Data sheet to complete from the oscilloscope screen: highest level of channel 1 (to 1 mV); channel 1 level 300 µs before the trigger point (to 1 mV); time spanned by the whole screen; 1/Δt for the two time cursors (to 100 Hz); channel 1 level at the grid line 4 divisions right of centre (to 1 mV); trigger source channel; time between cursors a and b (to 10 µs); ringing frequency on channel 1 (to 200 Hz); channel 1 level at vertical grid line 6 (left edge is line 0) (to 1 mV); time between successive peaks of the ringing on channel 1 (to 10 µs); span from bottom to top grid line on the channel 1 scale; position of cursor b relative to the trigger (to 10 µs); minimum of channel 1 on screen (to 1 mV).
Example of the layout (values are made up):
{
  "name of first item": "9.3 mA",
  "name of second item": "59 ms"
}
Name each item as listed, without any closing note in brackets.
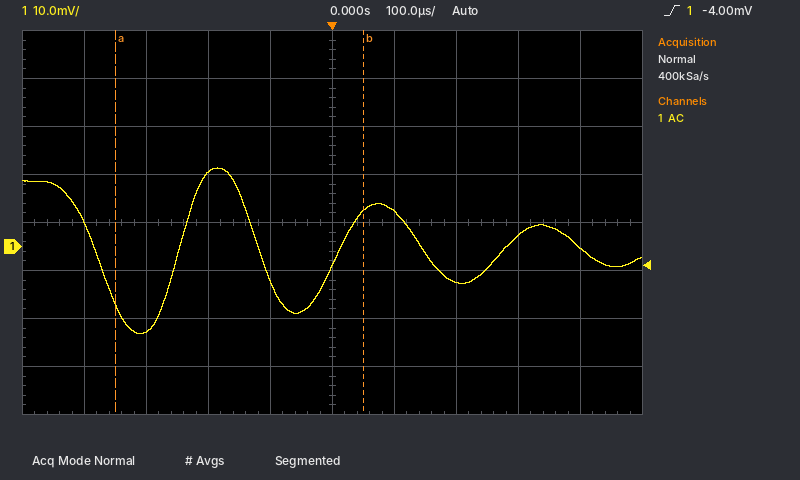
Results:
{
  "highest level of channel 1": "16 mV",
  "channel 1 level 300 µs before the trigger point": "-18 mV",
  "time spanned by the whole screen": "1 ms",
  "1/Δt for the two time cursors": "2.5 kHz",
  "channel 1 level at the grid line 4 divisions right of centre": "0 mV",
  "trigger source channel": "channel 1",
  "time between cursors a and b": "400 µs",
  "ringing frequency on channel 1": "3.8 kHz",
  "channel 1 level at vertical grid line 6 (left edge is line 0)": "7 mV",
  "time between successive peaks of the ringing on channel 1": "260 µs",
  "span from bottom to top grid line on the channel 1 scale": "80 mV",
  "position of cursor b relative to the trigger": "+50 µs",
  "minimum of channel 1 on screen": "-18 mV"
}
